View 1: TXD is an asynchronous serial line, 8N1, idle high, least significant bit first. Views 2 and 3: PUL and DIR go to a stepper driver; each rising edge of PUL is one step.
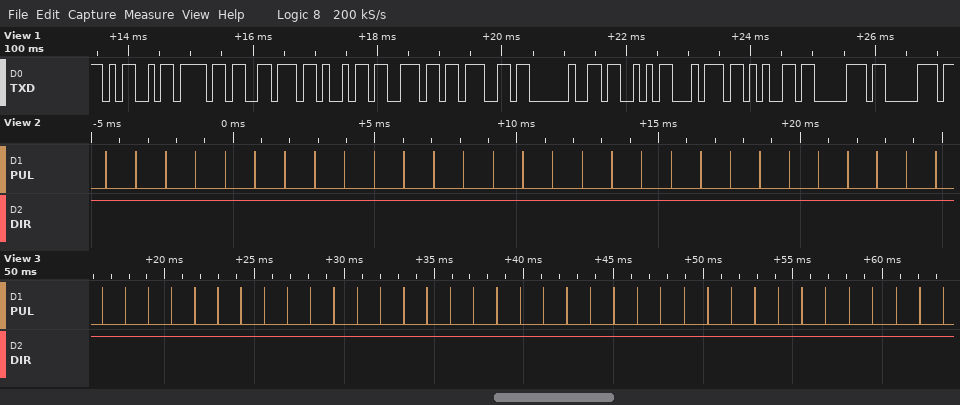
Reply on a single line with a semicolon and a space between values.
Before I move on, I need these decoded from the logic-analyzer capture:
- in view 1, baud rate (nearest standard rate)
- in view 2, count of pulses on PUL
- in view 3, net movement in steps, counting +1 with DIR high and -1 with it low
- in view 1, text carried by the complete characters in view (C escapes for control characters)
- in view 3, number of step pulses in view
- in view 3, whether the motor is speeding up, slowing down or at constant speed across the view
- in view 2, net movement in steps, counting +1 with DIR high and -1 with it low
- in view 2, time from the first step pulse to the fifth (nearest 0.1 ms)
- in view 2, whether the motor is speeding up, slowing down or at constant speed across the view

9600 baud; 29; +37; "Moving Stepp"; 37; constant speed; +29; 4.2 ms; constant speed
